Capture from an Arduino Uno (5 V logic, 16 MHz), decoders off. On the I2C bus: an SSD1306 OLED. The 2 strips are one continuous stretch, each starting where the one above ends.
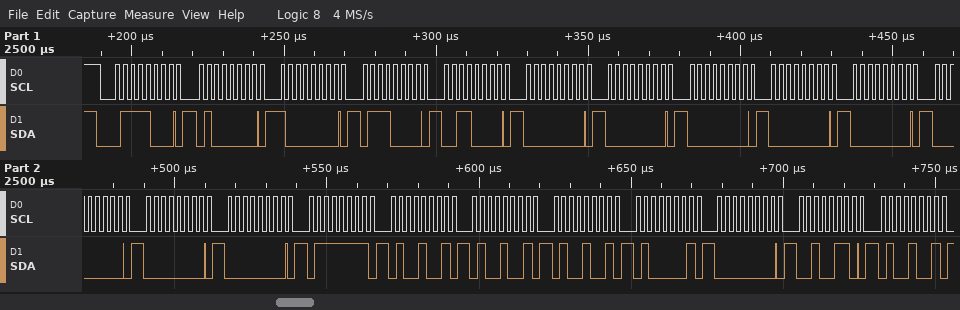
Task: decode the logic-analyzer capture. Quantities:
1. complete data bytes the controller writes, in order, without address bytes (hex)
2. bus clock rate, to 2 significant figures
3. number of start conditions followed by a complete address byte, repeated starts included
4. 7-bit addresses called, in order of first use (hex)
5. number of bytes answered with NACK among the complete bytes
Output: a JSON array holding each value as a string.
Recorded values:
["40 80 70 30 00 00 00 00 00 00 00 00 7F 49 49 49 41 00 26 49", "400 kHz", "1", "0x3C", "0"]
